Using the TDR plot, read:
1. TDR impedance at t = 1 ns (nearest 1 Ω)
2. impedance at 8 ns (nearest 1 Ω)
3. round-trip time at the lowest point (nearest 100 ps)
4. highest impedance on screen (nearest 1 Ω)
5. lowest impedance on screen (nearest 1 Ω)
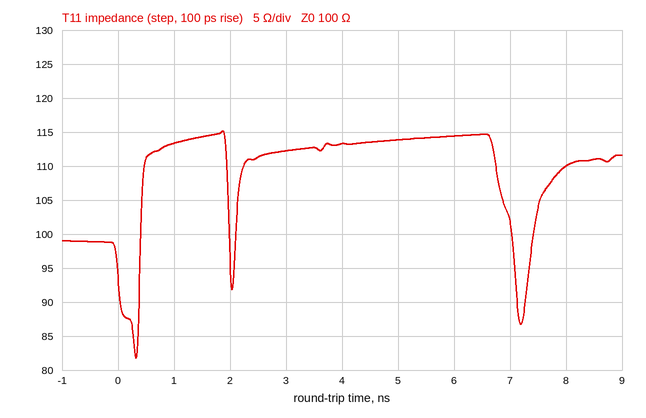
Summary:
113 Ω
110 Ω
300 ps
115 Ω
82 Ω
